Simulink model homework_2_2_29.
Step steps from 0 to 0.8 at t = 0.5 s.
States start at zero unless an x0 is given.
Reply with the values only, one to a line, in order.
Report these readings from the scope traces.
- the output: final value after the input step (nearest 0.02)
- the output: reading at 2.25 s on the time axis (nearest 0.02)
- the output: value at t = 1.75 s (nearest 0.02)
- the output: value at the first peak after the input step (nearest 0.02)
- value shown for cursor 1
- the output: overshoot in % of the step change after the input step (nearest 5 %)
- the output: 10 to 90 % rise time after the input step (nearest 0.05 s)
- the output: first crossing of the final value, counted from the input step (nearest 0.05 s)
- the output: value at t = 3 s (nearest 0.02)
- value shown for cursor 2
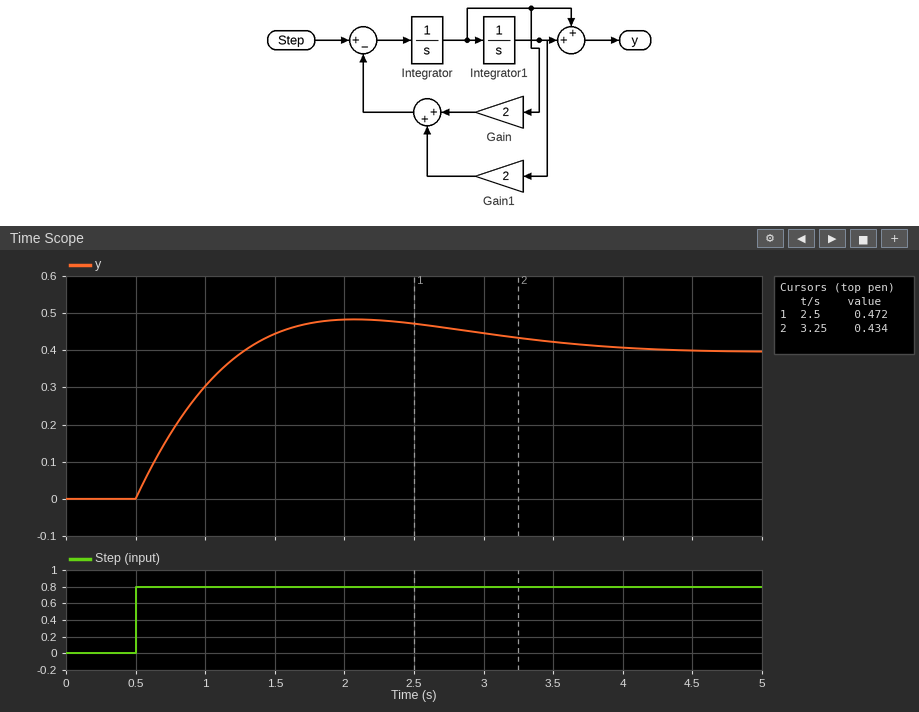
0.40
0.48
0.48
0.48
0.472
20 %
0.60 s
0.80 s
0.44
0.434
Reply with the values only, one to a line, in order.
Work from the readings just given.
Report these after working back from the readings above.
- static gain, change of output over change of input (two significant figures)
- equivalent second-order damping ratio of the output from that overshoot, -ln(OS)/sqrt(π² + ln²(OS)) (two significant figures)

0.50
0.46
